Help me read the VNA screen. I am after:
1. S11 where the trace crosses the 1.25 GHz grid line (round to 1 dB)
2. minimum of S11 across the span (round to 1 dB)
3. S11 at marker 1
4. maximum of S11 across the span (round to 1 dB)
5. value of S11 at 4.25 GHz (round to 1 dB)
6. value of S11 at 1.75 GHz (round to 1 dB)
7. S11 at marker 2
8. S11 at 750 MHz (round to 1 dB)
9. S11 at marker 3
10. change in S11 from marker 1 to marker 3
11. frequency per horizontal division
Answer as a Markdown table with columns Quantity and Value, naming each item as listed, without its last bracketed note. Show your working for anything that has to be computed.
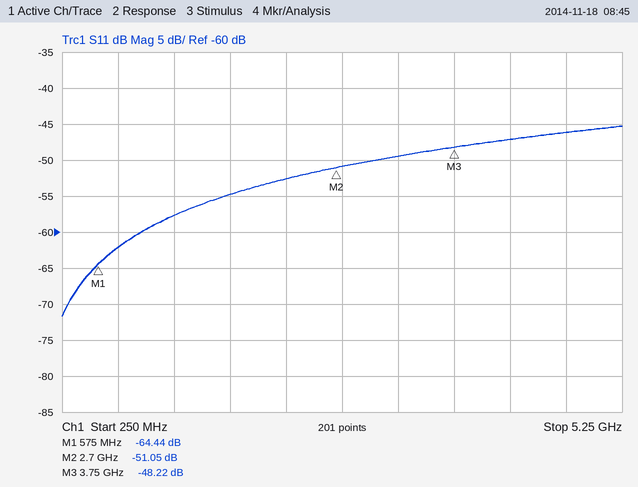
| Quantity | Value |
|---|---|
| S11 where the trace crosses the 1.25 GHz grid line | -58 dB |
| minimum of S11 across the span | -72 dB |
| S11 at marker 1 | -64.44 dB |
| maximum of S11 across the span | -45 dB |
| value of S11 at 4.25 GHz | -47 dB |
| value of S11 at 1.75 GHz | -55 dB |
| S11 at marker 2 | -51.05 dB |
| S11 at 750 MHz | -62 dB |
| S11 at marker 3 | -48.22 dB |
| change in S11 from marker 1 to marker 3 | -48.22 − (-64.44) = 16.22 dB |
| frequency per horizontal division | 500 MHz |
